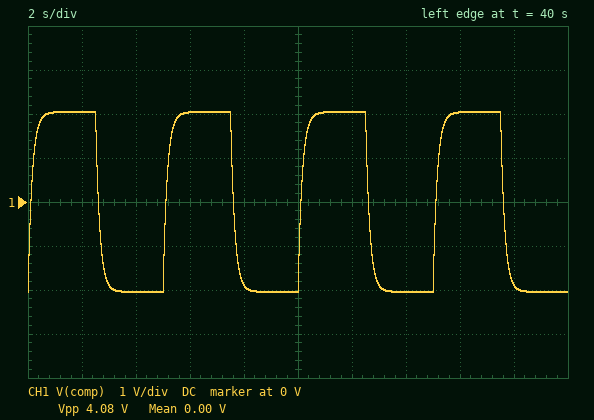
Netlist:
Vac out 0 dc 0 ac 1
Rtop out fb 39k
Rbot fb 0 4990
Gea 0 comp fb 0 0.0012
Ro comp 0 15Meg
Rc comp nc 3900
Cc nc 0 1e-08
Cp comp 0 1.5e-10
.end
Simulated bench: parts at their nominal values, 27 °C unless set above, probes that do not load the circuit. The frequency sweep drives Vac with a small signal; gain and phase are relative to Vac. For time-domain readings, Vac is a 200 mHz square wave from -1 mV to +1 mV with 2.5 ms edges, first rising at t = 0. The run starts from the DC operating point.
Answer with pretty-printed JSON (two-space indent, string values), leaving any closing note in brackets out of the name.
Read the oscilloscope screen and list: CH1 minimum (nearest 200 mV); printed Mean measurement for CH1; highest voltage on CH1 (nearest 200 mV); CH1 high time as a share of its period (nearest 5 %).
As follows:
{
  "CH1 minimum": "-2.0 V",
  "printed Mean measurement for CH1": "0.00 V",
  "highest voltage on CH1": "2.0 V",
  "CH1 high time as a share of its period": "50 %"
}
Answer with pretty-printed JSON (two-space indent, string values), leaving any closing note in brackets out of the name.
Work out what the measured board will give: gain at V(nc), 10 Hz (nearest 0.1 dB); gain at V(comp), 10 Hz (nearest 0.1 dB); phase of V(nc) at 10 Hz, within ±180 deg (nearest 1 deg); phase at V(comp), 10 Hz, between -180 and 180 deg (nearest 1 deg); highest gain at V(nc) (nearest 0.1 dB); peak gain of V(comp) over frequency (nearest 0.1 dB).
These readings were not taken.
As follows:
{
  "gain at V(nc), 10 Hz": "46.5 dB",
  "gain at V(comp), 10 Hz": "46.5 dB",
  "phase of V(nc) at 10 Hz, within ±180 deg": "-84 deg",
  "phase at V(comp), 10 Hz, between -180 and 180 deg": "-84 deg",
  "highest gain at V(nc)": "66.2 dB",
  "peak gain of V(comp) over frequency": "66.2 dB"
}
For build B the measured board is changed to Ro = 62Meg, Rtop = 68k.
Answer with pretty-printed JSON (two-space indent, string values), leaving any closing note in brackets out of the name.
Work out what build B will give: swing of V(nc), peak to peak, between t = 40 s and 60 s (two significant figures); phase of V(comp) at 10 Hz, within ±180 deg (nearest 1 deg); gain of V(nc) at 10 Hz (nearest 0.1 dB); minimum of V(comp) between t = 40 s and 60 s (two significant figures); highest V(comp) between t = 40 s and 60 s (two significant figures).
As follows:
{
  "swing of V(nc), peak to peak, between t = 40 s and 60 s": "9.8 V",
  "phase of V(comp) at 10 Hz, within ±180 deg": "-88 deg",
  "gain of V(nc) at 10 Hz": "42.2 dB",
  "minimum of V(comp) between t = 40 s and 60 s": "-4.9 V",
  "highest V(comp) between t = 40 s and 60 s": "4.9 V"
}
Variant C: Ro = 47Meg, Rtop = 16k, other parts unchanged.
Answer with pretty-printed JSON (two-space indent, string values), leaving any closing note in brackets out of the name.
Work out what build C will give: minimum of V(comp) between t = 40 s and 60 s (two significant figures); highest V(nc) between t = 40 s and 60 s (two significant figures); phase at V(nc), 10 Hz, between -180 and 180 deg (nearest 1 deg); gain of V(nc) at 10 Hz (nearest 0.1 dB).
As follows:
{
  "minimum of V(comp) between t = 40 s and 60 s": "-13 V",
  "highest V(nc) between t = 40 s and 60 s": "13 V",
  "phase at V(nc), 10 Hz, between -180 and 180 deg": "-88 deg",
  "gain of V(nc) at 10 Hz": "53.0 dB"
}
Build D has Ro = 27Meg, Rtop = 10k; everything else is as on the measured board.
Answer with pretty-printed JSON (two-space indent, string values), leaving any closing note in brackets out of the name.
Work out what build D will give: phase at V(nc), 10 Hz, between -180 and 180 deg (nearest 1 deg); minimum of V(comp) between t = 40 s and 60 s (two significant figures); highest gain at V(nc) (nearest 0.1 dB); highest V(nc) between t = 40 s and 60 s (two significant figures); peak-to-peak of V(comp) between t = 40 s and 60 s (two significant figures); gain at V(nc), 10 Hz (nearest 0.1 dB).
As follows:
{
  "phase at V(nc), 10 Hz, between -180 and 180 deg": "-87 deg",
  "minimum of V(comp) between t = 40 s and 60 s": "-11 V",
  "highest gain at V(nc)": "80.7 dB",
  "highest V(nc) between t = 40 s and 60 s": "11 V",
  "peak-to-peak of V(comp) between t = 40 s and 60 s": "22 V",
  "gain at V(nc), 10 Hz": "55.9 dB"
}
